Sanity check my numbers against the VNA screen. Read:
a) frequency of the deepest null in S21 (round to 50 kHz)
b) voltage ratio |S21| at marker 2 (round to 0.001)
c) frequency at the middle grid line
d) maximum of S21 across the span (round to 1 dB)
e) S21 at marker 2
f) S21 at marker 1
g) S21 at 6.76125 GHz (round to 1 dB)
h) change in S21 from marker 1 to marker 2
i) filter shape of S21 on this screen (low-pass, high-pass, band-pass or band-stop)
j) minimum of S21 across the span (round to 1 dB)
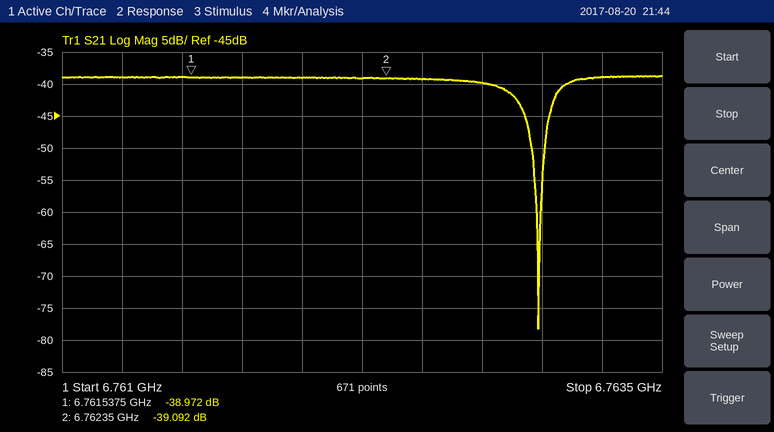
6.76300 GHz
0.011
6.76225 GHz
-39 dB
-39.092 dB
-38.972 dB
-39 dB
-0.120 dB
band-stop
-78 dB
